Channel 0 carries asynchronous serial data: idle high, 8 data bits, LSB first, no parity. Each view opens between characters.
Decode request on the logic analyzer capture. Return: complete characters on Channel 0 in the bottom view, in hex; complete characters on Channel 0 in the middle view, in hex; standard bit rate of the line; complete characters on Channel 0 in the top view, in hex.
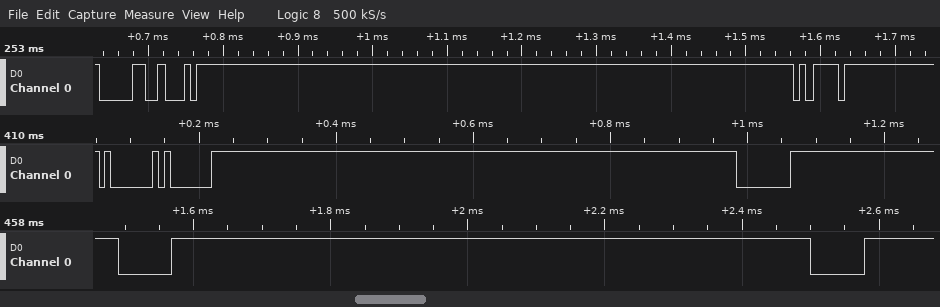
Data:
00, 00
01, 01, 00
115200 baud
30, F4, BD
